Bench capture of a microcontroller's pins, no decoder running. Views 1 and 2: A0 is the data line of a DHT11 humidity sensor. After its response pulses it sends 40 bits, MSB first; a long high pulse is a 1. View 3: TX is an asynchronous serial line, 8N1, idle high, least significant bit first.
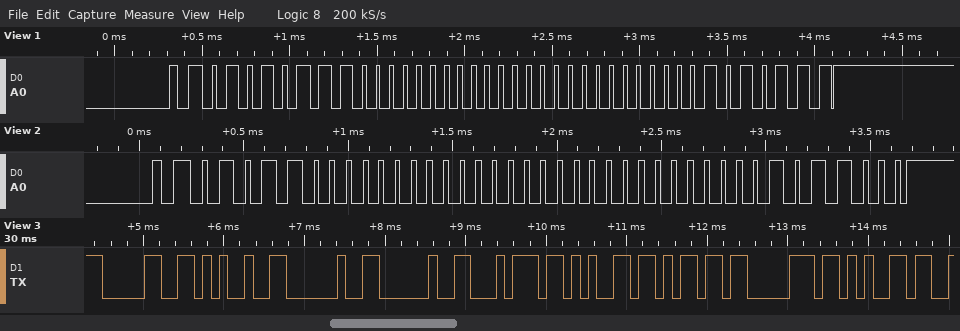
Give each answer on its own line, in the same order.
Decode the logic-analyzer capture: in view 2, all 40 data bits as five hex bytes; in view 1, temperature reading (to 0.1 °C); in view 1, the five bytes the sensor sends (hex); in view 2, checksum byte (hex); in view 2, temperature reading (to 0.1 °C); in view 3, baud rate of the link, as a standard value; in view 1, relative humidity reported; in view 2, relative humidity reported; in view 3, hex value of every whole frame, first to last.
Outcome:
58 00 00 00 58
0.0 °C
57 00 00 00 57
0x58
0.0 °C
9600 baud
87 %
88 %
30 25 20 20 74 65 6D 70 65
